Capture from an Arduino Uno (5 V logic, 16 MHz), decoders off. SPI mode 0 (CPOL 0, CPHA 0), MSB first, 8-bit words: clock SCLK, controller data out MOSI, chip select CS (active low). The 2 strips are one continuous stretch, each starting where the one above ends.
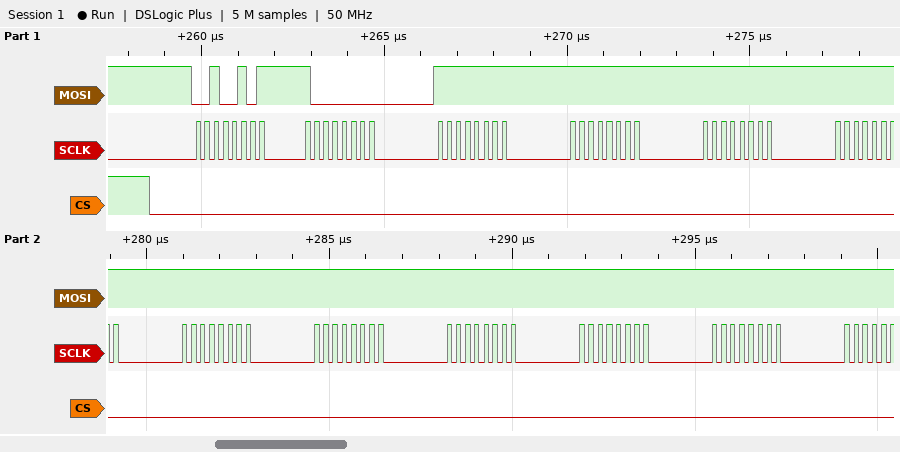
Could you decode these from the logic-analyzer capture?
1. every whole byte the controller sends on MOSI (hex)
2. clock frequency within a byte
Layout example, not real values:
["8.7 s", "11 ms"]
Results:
["0x25 0x80 0xFF 0xFF 0xFF 0xFF 0xFF 0xFF 0xFF 0xFF 0xFF", "4 MHz"]
